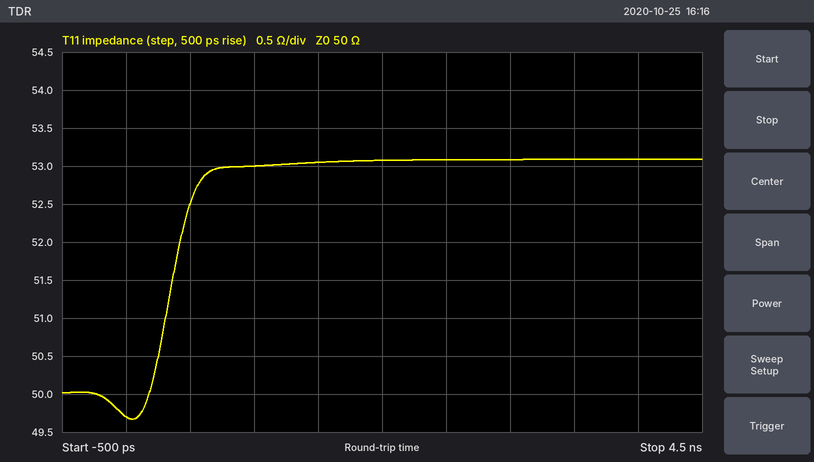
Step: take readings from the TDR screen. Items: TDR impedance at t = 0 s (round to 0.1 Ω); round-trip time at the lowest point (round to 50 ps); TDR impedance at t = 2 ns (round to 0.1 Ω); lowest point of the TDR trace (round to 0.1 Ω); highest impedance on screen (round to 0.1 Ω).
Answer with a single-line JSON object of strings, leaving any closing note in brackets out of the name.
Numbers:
{"TDR impedance at t = 0 s": "49.7 Ω", "round-trip time at the lowest point": "50 ps", "TDR impedance at t = 2 ns": "53.1 Ω", "lowest point of the TDR trace": "49.7 Ω", "highest impedance on screen": "53.1 Ω"}
